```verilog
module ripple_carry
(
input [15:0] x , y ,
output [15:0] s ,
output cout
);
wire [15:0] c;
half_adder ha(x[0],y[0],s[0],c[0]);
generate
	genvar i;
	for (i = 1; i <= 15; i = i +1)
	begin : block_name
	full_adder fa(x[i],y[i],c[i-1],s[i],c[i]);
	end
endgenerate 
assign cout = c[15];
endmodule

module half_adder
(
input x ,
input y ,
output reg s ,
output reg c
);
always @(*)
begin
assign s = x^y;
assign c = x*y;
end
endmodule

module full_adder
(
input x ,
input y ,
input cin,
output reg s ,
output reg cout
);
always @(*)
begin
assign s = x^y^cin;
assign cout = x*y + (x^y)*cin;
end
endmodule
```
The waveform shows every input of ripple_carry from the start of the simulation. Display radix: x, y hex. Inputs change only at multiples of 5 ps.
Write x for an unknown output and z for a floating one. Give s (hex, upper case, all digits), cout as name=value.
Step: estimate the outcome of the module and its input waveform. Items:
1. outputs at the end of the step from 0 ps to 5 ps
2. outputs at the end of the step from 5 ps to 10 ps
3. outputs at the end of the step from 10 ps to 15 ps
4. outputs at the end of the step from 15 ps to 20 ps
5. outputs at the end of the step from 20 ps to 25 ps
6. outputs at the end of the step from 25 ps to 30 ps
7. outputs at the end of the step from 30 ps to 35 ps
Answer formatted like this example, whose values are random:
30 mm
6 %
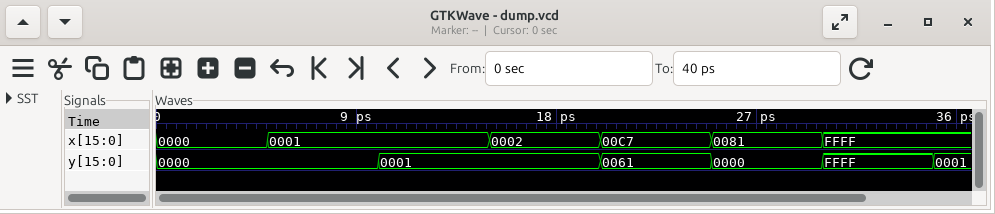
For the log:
s=0000, cout=0
s=0001, cout=0
s=0002, cout=0
s=0003, cout=0
s=0128, cout=0
s=0081, cout=0
s=FFFE, cout=1
